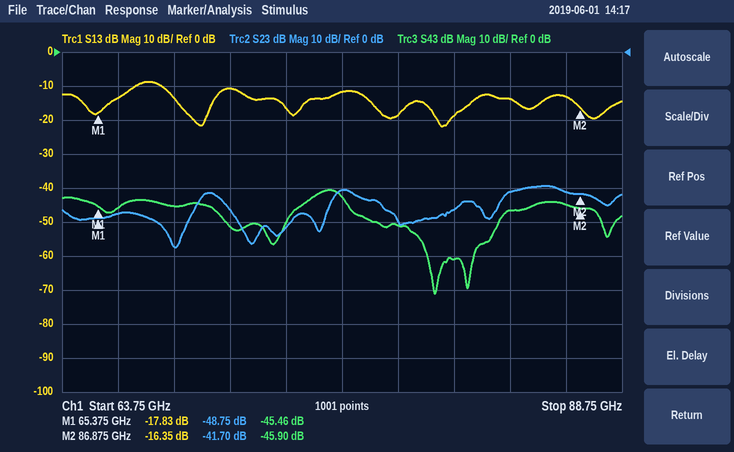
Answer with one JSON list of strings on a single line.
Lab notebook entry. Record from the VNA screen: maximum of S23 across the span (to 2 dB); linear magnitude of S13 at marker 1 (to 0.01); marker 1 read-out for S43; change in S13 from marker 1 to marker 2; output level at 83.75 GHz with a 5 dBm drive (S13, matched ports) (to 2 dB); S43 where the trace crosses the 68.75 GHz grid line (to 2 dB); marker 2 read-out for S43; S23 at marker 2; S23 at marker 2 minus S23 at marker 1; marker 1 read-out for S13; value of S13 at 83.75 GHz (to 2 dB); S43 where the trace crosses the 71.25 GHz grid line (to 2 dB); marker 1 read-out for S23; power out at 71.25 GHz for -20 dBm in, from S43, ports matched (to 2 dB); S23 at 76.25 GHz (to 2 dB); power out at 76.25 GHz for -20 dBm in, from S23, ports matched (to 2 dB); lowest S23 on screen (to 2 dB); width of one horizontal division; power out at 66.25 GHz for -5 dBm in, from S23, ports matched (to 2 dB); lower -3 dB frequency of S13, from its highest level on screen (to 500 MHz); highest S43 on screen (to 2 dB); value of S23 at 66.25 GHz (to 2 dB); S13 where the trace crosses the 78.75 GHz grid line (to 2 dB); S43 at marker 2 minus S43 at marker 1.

["-40 dB", "0.13", "-45.46 dB", "1.48 dB", "-8 dBm", "-46 dB", "-45.90 dB", "-41.70 dB", "7.05 dB", "-17.83 dB", "-14 dB", "-52 dB", "-48.75 dB", "-72 dBm", "-40 dB", "-60 dBm", "-58 dB", "2.5 GHz", "-52 dBm", "66.5 GHz", "-40 dB", "-48 dB", "-18 dB", "-0.44 dB"]
